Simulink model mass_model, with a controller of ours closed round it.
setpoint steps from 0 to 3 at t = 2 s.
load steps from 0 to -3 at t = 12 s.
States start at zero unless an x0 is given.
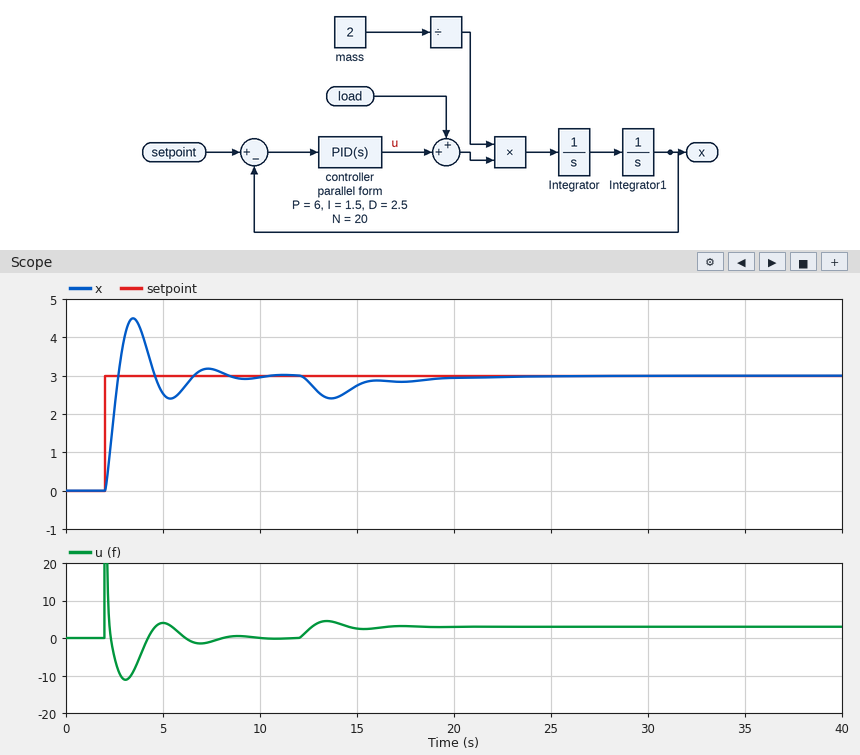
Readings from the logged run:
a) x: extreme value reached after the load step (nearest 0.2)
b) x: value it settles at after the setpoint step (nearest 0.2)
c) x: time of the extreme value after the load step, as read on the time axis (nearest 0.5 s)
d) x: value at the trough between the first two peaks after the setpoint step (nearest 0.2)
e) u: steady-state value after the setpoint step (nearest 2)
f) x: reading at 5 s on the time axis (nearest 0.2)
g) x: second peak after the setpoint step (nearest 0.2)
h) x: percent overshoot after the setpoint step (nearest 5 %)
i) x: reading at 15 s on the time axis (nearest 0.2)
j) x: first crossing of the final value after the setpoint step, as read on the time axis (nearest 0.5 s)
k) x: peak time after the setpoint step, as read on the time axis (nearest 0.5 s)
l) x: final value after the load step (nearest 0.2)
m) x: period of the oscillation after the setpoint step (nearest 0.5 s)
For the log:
2.4
3.0
13.5 s
2.4
0
2.6
3.2
50 %
2.8
2.5 s
3.5 s
3.0
4.0 s
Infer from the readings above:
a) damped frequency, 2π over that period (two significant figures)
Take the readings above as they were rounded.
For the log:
1.6 rad/s
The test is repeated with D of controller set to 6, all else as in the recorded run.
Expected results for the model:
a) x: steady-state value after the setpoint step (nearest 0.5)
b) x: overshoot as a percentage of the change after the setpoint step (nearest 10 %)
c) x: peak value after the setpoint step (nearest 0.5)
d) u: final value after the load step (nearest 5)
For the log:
3.0
20 %
3.5
5
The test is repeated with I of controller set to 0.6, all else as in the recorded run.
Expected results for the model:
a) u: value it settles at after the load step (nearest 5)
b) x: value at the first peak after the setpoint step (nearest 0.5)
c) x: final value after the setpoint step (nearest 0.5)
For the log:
5
4.5
3.0
